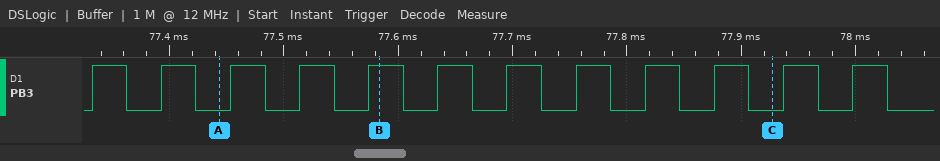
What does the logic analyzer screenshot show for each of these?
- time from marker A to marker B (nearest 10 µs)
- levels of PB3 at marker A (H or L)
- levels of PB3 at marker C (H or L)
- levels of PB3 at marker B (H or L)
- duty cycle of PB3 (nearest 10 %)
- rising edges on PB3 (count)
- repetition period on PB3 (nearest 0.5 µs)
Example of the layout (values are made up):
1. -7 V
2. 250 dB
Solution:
1. 140 µs
2. PB3=L
3. PB3=L
4. PB3=H
5. 50 %
6. 12
7. 60.5 µs
